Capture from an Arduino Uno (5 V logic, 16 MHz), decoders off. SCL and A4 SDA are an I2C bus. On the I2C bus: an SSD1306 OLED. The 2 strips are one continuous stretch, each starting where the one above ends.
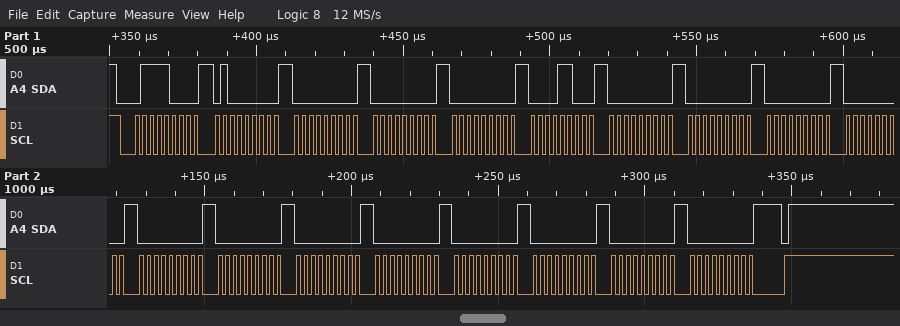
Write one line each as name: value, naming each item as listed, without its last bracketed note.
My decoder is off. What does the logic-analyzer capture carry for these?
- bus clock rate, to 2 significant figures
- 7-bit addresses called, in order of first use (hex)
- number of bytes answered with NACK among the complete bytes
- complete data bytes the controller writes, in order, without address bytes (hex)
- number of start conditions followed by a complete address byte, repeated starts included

bus clock rate, to 2 significant figures: 400 kHz
7-bit addresses called, in order of first use: 0x3C
number of bytes answered with NACK among the complete bytes: 0
complete data bytes the controller writes, in order, without address bytes: 40 00 00 00 0C 00 00 00 00 00 00 00 00 00 00 00 00
number of start conditions followed by a complete address byte, repeated starts included: 1
